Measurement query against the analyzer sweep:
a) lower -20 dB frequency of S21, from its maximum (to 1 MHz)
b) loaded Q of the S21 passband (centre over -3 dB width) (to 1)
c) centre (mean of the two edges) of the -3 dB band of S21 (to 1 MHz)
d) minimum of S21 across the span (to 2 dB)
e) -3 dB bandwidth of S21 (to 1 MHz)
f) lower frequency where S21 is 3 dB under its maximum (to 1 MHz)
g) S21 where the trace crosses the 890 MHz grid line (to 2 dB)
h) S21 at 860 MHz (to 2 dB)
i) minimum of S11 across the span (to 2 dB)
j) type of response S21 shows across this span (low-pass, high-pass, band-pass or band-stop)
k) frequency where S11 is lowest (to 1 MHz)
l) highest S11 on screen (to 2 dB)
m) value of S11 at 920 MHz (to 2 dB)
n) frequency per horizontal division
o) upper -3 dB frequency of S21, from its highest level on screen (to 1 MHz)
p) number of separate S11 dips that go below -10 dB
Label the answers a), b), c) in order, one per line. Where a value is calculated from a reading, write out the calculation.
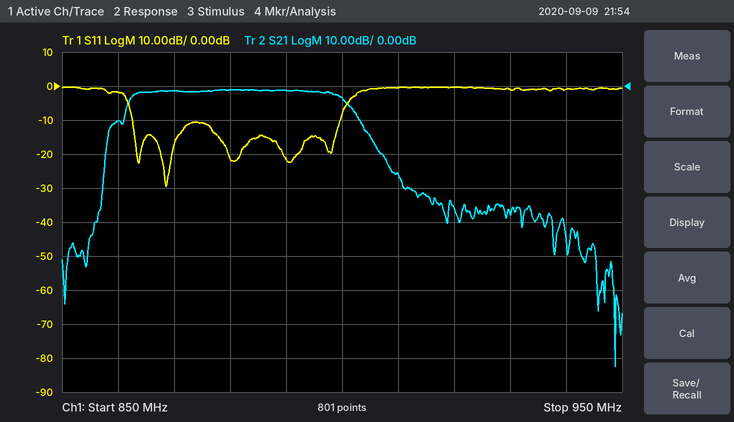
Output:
a) 858 MHz
b) 881 MHz / 38 MHz ≈ 23
c) 881 MHz
d) -82 dB
e) 900 MHz − 862 MHz = 38 MHz
f) 862 MHz
g) -2 dB
h) -10 dB
i) -30 dB
j) band-pass
k) 869 MHz
l) 0 dB
m) 0 dB
n) 10 MHz
o) 900 MHz
p) 5
